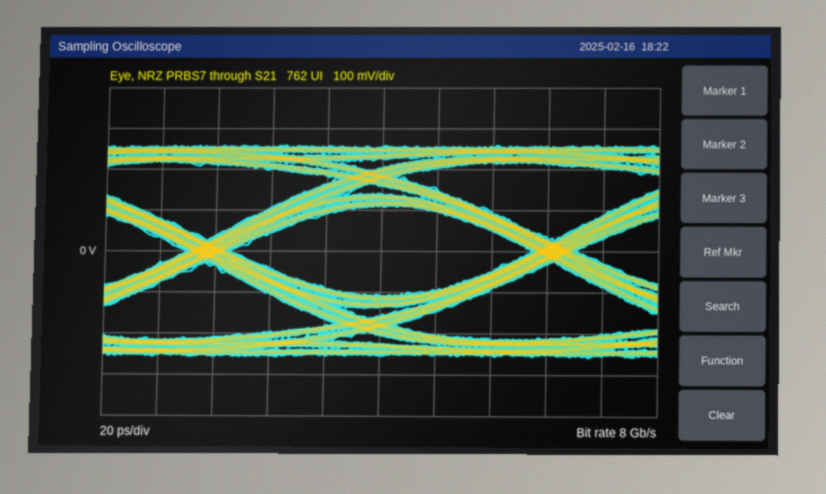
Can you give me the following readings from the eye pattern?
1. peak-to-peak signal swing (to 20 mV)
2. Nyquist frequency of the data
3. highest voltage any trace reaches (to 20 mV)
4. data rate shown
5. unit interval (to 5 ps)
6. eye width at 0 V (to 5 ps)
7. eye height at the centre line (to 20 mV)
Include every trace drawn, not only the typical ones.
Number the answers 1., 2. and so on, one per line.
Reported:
1. 520 mV
2. 4 GHz
3. 260 mV
4. 8 Gb/s
5. 125 ps
6. 110 ps
7. 220 mV
